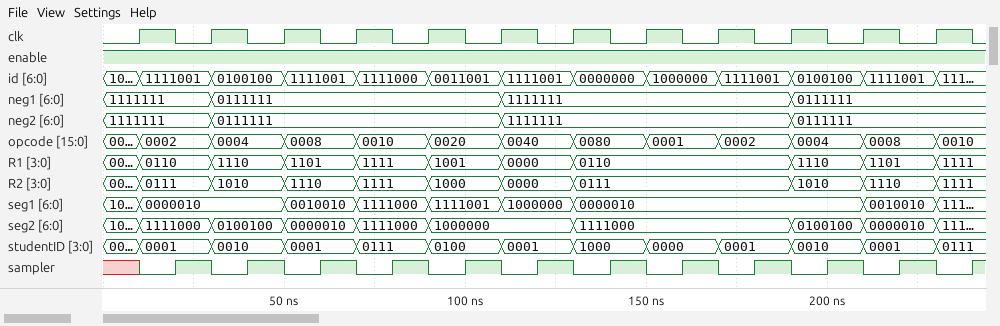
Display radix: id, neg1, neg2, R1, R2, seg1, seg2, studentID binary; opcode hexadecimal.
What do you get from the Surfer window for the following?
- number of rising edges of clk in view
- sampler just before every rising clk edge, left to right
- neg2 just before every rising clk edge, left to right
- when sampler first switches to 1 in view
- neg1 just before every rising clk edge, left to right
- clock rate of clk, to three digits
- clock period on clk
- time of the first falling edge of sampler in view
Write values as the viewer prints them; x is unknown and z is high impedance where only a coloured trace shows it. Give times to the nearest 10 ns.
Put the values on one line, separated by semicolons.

12; x 1 1 1 1 1 1 1 1 1 1 1; 1111111, 1111111, 0111111, 0111111, 0111111, 0111111, 1111111, 1111111, 1111111, 1111111, 0111111, 0111111; 20 ns; 1111111, 1111111, 0111111, 0111111, 0111111, 0111111, 1111111, 1111111, 1111111, 1111111, 0111111, 0111111; 50.0 MHz; 20 ns; 30 ns
